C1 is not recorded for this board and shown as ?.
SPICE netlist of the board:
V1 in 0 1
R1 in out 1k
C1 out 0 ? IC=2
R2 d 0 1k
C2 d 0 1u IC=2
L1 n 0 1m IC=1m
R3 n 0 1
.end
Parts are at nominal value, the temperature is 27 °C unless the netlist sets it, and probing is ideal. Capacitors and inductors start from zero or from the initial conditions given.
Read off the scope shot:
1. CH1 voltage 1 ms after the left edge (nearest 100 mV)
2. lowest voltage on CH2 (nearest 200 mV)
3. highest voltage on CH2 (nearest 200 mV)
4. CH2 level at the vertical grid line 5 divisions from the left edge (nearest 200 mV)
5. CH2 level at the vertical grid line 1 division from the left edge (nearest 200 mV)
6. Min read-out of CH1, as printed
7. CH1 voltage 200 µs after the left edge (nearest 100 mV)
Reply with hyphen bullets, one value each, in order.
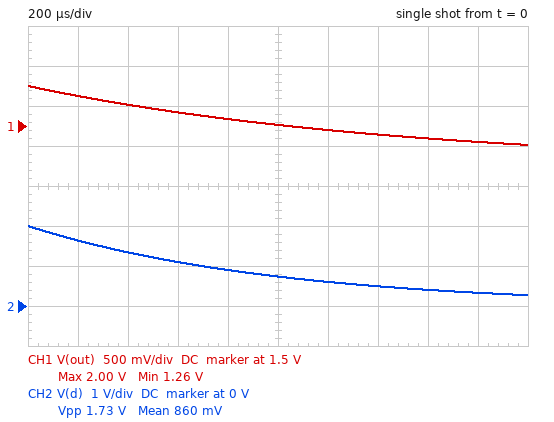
- 1.5 V
- 200 mV
- 2.0 V
- 800 mV
- 1.6 V
- 1.26 V
- 1.9 V
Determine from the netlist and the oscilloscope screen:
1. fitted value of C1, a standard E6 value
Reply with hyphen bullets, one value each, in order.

- 1.5 µF
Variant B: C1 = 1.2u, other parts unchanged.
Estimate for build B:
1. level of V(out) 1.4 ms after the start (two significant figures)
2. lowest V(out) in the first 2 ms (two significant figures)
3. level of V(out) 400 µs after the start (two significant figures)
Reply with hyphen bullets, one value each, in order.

- 1.3 V
- 1.2 V
- 1.7 V
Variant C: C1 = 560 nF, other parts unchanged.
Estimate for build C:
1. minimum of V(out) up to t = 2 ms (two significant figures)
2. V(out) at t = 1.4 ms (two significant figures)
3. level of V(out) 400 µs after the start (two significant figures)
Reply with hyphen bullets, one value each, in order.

- 1.0 V
- 1.1 V
- 1.5 V
